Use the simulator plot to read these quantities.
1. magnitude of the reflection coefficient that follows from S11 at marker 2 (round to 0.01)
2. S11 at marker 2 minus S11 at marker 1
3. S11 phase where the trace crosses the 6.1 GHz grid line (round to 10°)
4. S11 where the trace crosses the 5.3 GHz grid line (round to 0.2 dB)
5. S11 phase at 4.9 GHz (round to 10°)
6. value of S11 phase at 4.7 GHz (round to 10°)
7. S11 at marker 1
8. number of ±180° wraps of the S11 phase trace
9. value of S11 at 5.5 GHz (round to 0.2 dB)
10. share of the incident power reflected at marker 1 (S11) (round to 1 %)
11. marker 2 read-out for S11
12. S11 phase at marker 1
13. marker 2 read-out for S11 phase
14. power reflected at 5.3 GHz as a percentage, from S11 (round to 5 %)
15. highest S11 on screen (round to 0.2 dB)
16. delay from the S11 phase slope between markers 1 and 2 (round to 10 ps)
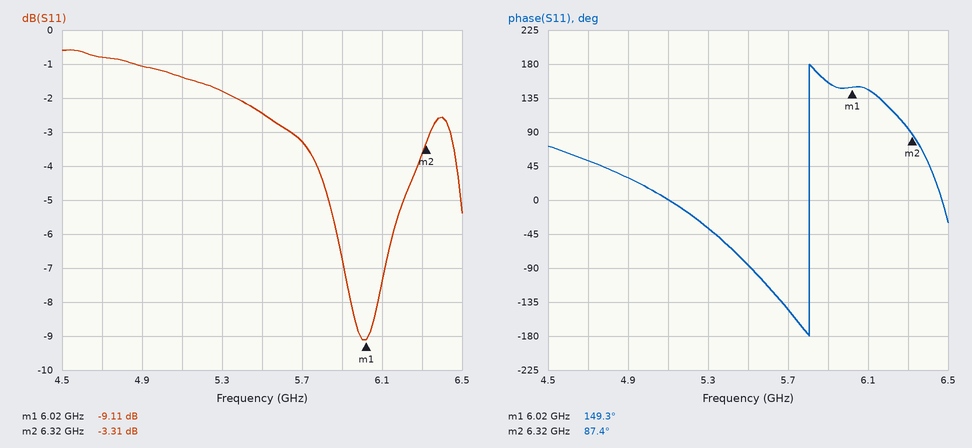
0.68
5.80 dB
150°
-1.8 dB
30°
50°
-9.11 dB
1
-2.4 dB
12 %
-3.31 dB
149.3°
87.4°
65 %
-0.6 dB
570 ps
